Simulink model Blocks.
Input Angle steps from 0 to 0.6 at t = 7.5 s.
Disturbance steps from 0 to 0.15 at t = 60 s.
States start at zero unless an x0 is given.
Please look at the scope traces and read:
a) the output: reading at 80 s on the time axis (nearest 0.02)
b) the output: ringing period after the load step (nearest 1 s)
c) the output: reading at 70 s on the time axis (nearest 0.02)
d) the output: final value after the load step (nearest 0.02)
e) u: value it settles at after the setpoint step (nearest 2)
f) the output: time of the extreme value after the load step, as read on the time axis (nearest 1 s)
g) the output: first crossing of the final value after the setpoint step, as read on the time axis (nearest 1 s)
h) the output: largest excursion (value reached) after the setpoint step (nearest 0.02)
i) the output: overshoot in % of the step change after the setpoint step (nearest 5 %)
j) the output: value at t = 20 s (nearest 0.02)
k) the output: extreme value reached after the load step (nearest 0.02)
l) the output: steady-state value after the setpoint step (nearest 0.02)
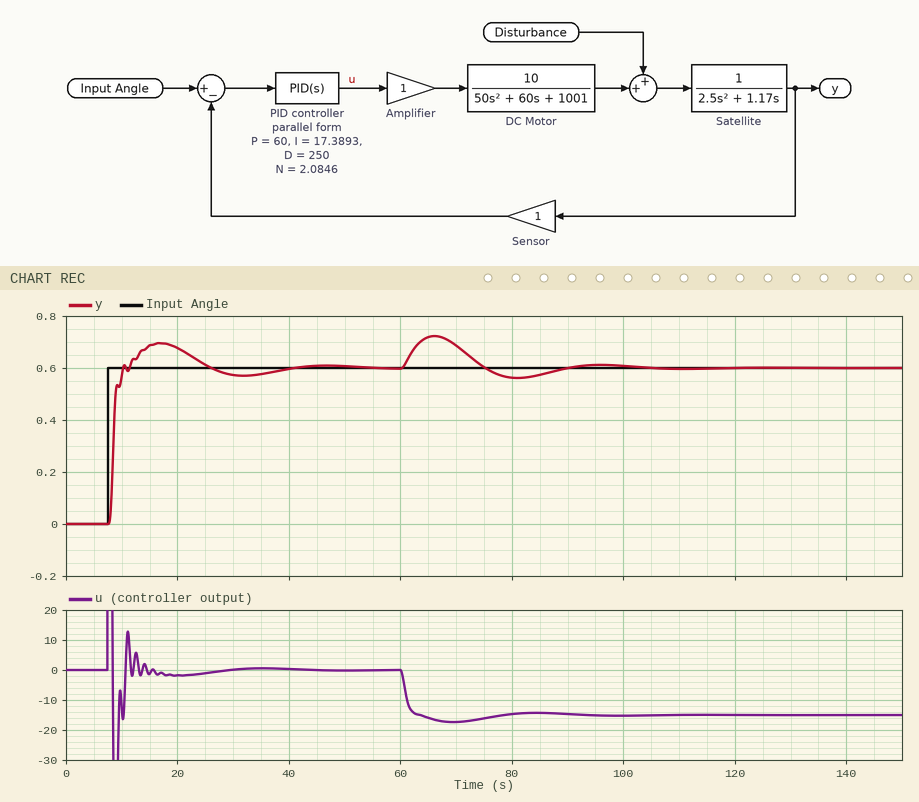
0.56
30 s
0.68
0.60
0
66 s
10 s
0.70
15 %
0.68
0.72
0.60
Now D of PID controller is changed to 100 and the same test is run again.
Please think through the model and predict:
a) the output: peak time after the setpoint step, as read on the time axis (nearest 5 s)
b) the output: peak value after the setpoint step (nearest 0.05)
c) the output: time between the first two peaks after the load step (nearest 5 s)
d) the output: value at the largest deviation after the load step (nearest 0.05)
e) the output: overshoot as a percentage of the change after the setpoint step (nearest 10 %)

15 s
0.80
20 s
0.75
30 %
